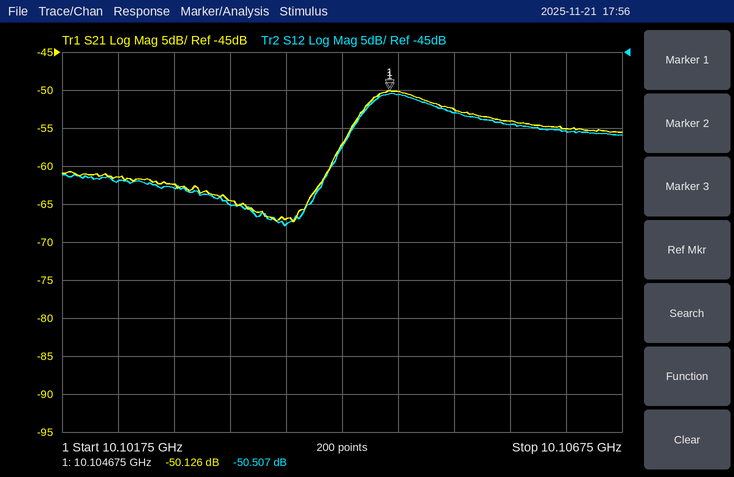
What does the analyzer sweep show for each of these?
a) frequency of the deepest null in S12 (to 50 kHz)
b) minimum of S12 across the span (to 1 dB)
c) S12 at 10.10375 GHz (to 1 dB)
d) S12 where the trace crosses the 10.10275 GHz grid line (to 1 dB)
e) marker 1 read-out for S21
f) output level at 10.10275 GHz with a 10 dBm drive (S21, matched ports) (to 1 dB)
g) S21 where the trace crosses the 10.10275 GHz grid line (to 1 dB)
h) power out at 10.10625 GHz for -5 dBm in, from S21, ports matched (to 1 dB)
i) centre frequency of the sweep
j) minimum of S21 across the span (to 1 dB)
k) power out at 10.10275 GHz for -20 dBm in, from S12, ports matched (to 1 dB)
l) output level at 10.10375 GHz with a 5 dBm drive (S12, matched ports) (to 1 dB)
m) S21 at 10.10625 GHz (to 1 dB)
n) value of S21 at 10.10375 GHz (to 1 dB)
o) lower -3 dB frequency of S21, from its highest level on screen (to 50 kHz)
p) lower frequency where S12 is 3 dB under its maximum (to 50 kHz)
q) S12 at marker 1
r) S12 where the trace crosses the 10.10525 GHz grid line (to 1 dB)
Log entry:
10.10375 GHz
-68 dB
-68 dB
-63 dB
-50.126 dB
-52 dBm
-62 dB
-60 dBm
10.10425 GHz
-67 dB
-83 dBm
-63 dBm
-55 dB
-67 dB
10.10440 GHz
10.10440 GHz
-50.507 dB
-53 dB
